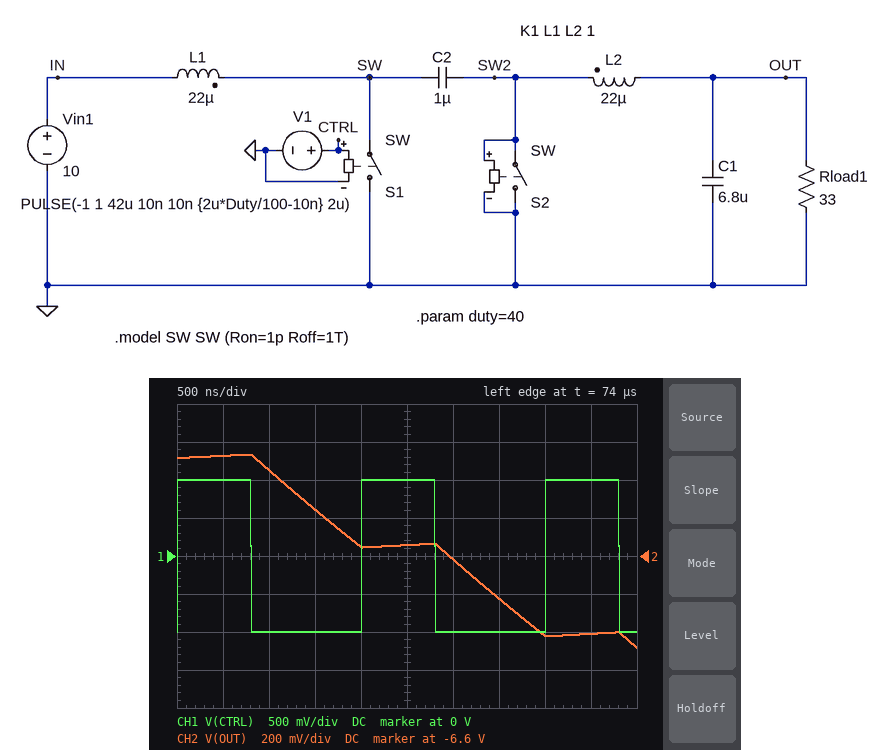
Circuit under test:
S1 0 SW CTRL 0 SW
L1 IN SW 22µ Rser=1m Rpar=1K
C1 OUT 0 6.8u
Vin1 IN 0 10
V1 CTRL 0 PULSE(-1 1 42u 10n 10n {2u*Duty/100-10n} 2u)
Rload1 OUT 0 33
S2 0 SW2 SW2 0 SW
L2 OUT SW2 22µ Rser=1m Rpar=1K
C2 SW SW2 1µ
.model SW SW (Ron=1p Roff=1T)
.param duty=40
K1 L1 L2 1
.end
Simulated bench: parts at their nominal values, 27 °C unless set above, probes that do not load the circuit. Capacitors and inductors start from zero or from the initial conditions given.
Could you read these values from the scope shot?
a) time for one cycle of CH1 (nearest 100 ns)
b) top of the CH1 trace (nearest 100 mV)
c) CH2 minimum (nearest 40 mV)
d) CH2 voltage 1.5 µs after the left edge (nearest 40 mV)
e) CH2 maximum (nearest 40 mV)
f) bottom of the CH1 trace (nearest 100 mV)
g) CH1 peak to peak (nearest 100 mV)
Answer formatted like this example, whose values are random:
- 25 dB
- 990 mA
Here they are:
- 2.0 µs
- 1.0 V
- -7.08 V
- -6.36 V
- -6.08 V
- -1.0 V
- 2.0 V
